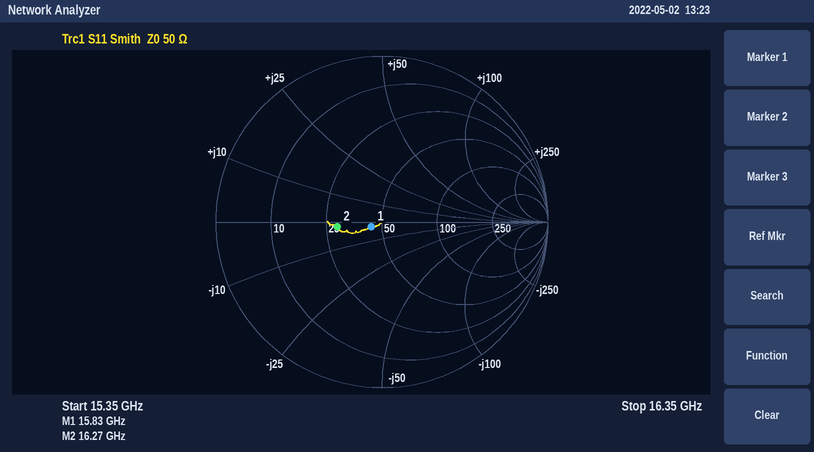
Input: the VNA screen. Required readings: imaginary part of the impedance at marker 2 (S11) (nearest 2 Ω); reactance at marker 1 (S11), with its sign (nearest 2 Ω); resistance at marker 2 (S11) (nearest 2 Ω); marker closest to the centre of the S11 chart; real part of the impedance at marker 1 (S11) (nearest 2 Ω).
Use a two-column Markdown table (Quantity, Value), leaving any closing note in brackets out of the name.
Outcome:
| Quantity | Value |
|---|---|
| imaginary part of the impedance at marker 2 (S11) | -2 Ω |
| reactance at marker 1 (S11), with its sign | -2 Ω |
| resistance at marker 2 (S11) | 28 Ω |
| marker closest to the centre of the S11 chart | marker 1 |
| real part of the impedance at marker 1 (S11) | 44 Ω |
